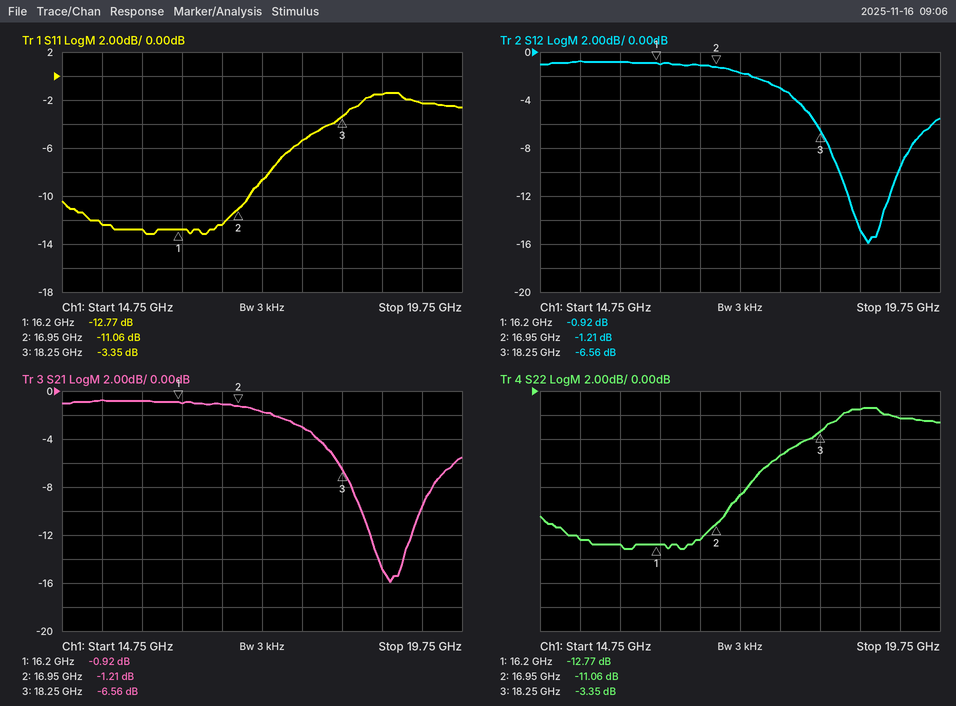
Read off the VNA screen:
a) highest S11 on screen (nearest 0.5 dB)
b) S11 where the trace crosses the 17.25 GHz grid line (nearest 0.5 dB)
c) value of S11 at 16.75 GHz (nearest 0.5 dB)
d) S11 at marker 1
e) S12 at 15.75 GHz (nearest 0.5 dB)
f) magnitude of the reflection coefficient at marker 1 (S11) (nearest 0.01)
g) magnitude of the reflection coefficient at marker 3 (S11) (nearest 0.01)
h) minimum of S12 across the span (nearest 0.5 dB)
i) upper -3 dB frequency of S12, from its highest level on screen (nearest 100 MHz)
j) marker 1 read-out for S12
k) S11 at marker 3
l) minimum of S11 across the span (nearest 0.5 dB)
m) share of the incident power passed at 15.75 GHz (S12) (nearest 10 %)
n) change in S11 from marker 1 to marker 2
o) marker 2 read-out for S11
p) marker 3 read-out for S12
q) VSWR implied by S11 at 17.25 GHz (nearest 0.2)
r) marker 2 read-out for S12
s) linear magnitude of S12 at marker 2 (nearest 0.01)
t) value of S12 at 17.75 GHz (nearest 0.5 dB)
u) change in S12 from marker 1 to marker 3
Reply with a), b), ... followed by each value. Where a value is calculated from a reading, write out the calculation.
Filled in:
a) -1.5 dB
b) -8.5 dB
c) -12.5 dB
d) -12.77 dB
e) -1.0 dB
f) 10^(-12.77/20) ≈ 0.23
g) 10^(-3.35/20) ≈ 0.68
h) -16.0 dB
i) 17.9 GHz
j) -0.92 dB
k) -3.35 dB
l) -13.0 dB
m) 10^(-1/10) ≈ 79.4 %, so 80 % to the nearest 10 %
n) -11.06 − (-12.77) = 1.71 dB
o) -11.06 dB
p) -6.56 dB
q) |Γ| = 10^(-8.5/20) = 0.3758; VSWR = (1 + 0.3758)/(1 − 0.3758) ≈ 2.2
r) -1.21 dB
s) 10^(-1.21/20) ≈ 0.87
t) -3.0 dB
u) -6.56 − (-0.92) = -5.64 dB
